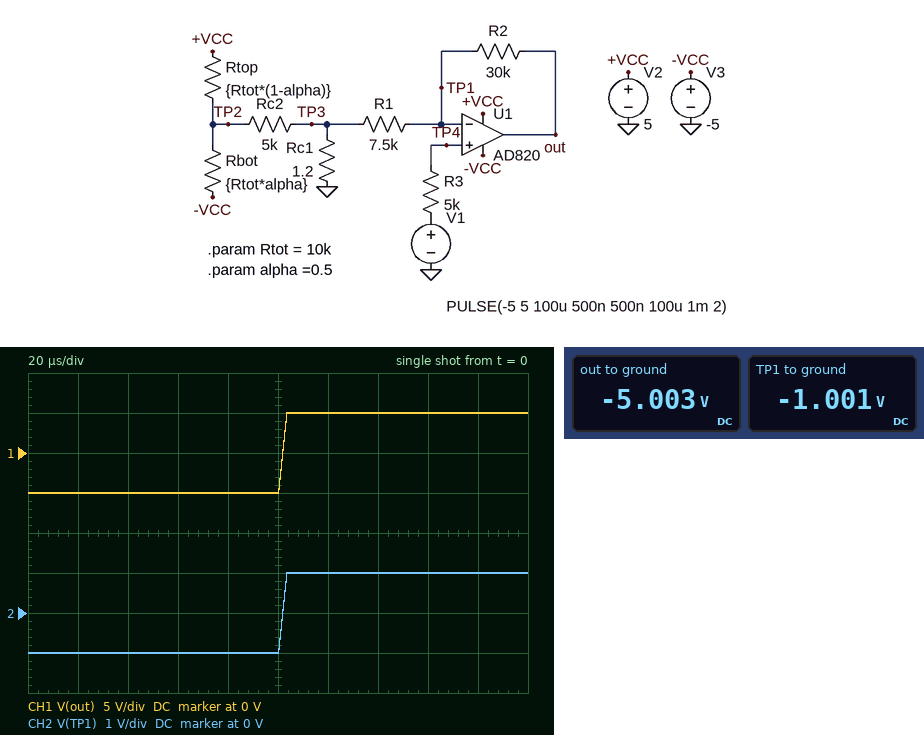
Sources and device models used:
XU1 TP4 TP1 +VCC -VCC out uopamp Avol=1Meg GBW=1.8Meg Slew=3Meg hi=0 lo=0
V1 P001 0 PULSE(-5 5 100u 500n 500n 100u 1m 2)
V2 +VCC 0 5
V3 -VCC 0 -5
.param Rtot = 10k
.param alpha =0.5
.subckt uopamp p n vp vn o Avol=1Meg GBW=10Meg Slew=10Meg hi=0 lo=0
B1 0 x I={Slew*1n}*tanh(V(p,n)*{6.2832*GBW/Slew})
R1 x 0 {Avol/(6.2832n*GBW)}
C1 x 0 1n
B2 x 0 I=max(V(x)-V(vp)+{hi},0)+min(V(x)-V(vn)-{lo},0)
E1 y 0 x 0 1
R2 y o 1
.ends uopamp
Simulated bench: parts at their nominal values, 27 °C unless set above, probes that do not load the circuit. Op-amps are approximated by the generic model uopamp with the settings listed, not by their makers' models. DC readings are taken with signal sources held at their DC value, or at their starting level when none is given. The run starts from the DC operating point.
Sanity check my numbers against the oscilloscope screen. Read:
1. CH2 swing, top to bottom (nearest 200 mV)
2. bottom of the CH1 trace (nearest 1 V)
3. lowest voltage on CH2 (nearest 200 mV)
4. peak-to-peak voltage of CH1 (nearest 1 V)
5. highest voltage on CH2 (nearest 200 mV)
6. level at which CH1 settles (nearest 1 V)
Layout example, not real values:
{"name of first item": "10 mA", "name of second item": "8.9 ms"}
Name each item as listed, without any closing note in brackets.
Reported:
{"CH2 swing, top to bottom": "2.0 V", "bottom of the CH1 trace": "-5 V", "lowest voltage on CH2": "-1.0 V", "peak-to-peak voltage of CH1": "10 V", "highest voltage on CH2": "1.0 V", "level at which CH1 settles": "5 V"}
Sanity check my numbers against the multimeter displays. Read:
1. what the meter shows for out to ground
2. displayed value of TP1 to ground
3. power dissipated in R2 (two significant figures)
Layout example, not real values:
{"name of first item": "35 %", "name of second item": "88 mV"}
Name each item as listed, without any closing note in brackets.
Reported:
{"what the meter shows for out to ground": "-5.003 V", "displayed value of TP1 to ground": "-1.001 V", "power dissipated in R2": "530 µW"}
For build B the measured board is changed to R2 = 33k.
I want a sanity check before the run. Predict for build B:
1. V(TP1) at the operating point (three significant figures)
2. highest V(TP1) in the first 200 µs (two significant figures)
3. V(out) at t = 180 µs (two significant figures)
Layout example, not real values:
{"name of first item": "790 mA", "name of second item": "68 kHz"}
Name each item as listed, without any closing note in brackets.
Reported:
{"V(TP1) at the operating point": "-927 mV", "highest V(TP1) in the first 200 µs": "930 mV", "V(out) at t = 180 µs": "5.0 V"}
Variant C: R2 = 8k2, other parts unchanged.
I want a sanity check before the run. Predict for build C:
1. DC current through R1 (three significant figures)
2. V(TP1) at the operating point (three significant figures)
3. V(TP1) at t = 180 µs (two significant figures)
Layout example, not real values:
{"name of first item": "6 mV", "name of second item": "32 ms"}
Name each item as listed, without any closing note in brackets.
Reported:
{"DC current through R1": "319 µA", "V(TP1) at the operating point": "-2.39 V", "V(TP1) at t = 180 µs": "2.4 V"}
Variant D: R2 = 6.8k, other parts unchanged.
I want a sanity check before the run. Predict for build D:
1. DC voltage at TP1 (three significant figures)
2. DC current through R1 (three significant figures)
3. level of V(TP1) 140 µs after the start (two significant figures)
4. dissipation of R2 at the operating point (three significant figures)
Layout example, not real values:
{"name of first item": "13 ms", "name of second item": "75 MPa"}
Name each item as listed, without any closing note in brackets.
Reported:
{"DC voltage at TP1": "-2.62 V", "DC current through R1": "350 µA", "level of V(TP1) 140 µs after the start": "2.6 V", "dissipation of R2 at the operating point": "832 µW"}
